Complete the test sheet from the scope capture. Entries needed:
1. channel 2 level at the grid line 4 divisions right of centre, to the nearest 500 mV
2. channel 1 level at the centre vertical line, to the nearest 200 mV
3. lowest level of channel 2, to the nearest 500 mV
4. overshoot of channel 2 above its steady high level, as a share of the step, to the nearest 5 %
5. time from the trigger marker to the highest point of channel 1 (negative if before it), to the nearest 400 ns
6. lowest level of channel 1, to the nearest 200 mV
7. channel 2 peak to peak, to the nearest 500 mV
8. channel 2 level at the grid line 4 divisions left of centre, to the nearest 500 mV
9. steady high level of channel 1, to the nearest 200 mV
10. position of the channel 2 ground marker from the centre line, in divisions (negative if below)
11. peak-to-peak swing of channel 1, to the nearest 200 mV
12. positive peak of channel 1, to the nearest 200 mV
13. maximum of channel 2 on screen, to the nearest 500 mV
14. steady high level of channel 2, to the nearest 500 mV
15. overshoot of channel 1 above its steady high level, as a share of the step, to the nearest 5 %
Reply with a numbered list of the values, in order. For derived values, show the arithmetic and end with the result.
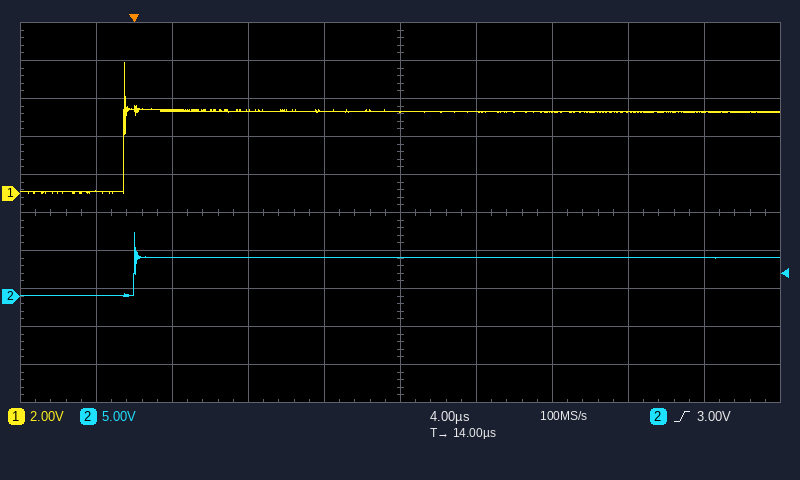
1. 5.0 V
2. 4.2 V
3. 0.0 V
4. 65 %
5. -400 ns
6. 0.0 V
7. 8.5 V − (0.0 V) = 8.5 V
8. 0.0 V
9. 4.4 V
10. -2.2 div
11. 6.8 V − (0.0 V) = 6.8 V
12. 6.8 V
13. 8.5 V
14. 5.0 V
15. 60 %
